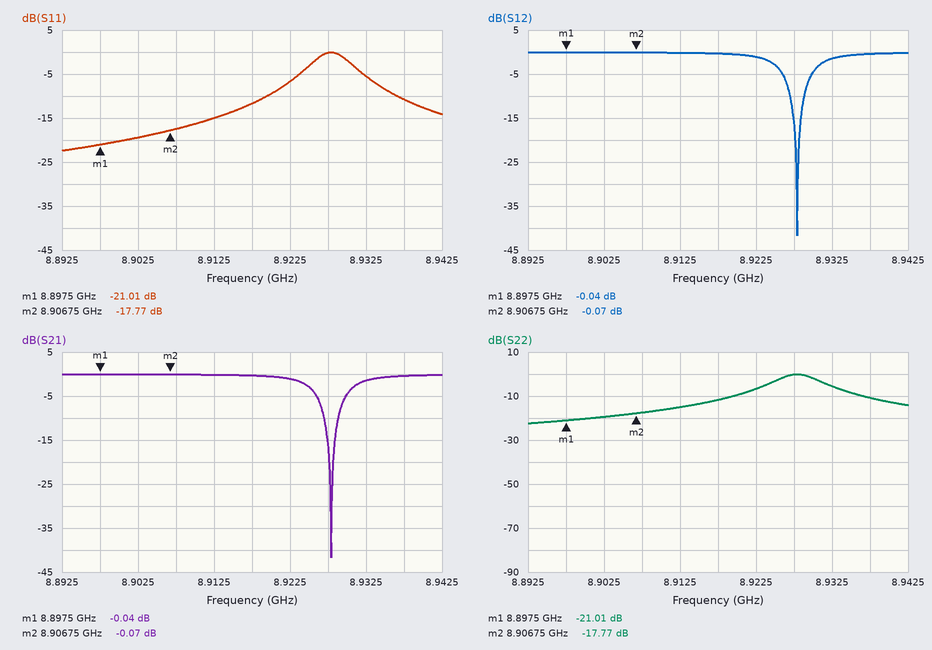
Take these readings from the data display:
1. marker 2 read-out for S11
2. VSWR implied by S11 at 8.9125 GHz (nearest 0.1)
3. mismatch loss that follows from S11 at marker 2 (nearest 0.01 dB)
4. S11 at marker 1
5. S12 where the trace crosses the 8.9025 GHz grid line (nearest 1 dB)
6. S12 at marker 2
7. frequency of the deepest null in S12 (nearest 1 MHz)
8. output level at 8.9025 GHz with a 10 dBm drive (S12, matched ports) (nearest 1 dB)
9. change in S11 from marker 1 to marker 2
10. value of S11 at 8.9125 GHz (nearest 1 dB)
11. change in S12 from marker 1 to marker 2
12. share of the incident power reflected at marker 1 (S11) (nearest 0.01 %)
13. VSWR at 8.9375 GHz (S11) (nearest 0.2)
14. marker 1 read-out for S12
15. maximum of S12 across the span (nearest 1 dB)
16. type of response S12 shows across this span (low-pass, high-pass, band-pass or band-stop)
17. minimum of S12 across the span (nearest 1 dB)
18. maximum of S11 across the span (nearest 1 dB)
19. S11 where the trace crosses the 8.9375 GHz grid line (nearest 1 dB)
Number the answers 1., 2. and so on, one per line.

1. -17.77 dB
2. 1.4
3. 0.07 dB
4. -21.01 dB
5. 0 dB
6. -0.07 dB
7. 8.928 GHz
8. 10 dBm
9. 3.24 dB
10. -15 dB
11. -0.03 dB
12. 0.79 %
13. 1.8
14. -0.04 dB
15. 0 dB
16. band-stop
17. -42 dB
18. 0 dB
19. -11 dB
